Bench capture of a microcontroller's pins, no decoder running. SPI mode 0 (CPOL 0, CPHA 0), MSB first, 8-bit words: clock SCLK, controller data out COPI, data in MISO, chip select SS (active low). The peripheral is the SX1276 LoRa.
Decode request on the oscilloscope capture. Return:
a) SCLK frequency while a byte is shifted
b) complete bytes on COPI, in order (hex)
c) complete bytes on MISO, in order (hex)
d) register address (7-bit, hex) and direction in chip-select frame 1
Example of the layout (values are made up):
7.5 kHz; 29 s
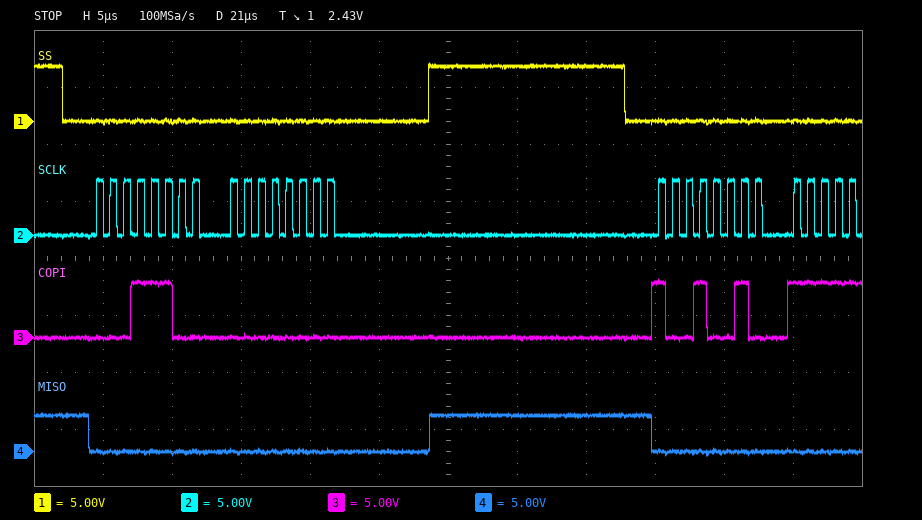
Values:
1 MHz; 1C 00 92; 00 00 00; 0x1C read
